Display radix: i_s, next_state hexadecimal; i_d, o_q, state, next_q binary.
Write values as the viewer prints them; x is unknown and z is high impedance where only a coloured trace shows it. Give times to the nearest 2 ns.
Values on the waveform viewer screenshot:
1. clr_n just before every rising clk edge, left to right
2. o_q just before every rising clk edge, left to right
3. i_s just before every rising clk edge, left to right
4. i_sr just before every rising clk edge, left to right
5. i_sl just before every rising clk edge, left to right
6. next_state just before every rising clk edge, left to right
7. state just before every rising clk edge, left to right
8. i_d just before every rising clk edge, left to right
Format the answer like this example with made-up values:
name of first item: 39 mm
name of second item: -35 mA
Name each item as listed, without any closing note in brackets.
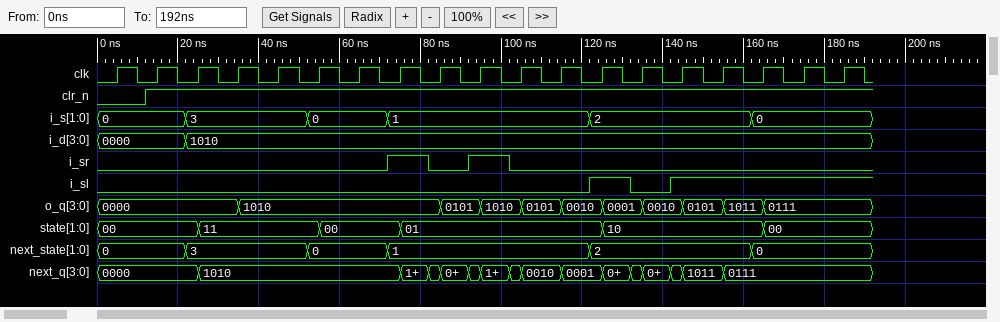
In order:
clr_n just before every rising clk edge, left to right: 0 1 1 1 1 1 1 1 1 1 1 1 1 1 1 1 1 1 1
o_q just before every rising clk edge, left to right: 0000, 0000, 0000, 0000, 1010, 1010, 1010, 1010, 1010, 0101, 1010, 0101, 0010, 0001, 0010, 0101, 1011, 0111, 0111
i_s just before every rising clk edge, left to right: 0, 0, 3, 3, 3, 0, 0, 1, 1, 1, 1, 1, 2, 2, 2, 2, 0, 0, 0
i_sr just before every rising clk edge, left to right: 0 0 0 0 0 0 0 1 0 1 0 0 0 0 0 0 0 0 0
i_sl just before every rising clk edge, left to right: 0 0 0 0 0 0 0 0 0 0 0 0 1 0 1 1 1 1 1
next_state just before every rising clk edge, left to right: 0, 0, 3, 3, 3, 0, 0, 1, 1, 1, 1, 1, 2, 2, 2, 2, 0, 0, 0
state just before every rising clk edge, left to right: 00, 00, 00, 11, 11, 11, 00, 00, 01, 01, 01, 01, 01, 10, 10, 10, 10, 00, 00
i_d just before every rising clk edge, left to right: 0000, 0000, 1010, 1010, 1010, 1010, 1010, 1010, 1010, 1010, 1010, 1010, 1010, 1010, 1010, 1010, 1010, 1010, 1010
